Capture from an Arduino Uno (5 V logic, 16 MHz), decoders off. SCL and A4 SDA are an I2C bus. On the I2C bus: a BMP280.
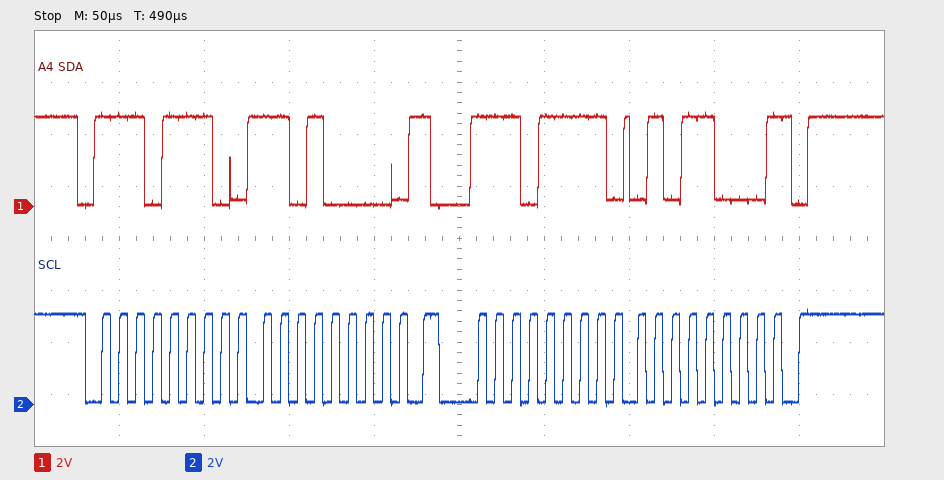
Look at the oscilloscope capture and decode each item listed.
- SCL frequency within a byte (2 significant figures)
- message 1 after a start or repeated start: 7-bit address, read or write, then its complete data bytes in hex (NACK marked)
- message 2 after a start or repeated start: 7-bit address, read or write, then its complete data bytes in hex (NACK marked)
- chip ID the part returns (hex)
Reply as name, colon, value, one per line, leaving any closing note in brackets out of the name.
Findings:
SCL frequency within a byte: 100 kHz
message 1 after a start or repeated start: 7-bit address, read or write, then its complete data bytes in hex: 0x77 write: D0
message 2 after a start or repeated start: 7-bit address, read or write, then its complete data bytes in hex: 0x77 read: 58 NACK
chip ID the part returns: 0x58
